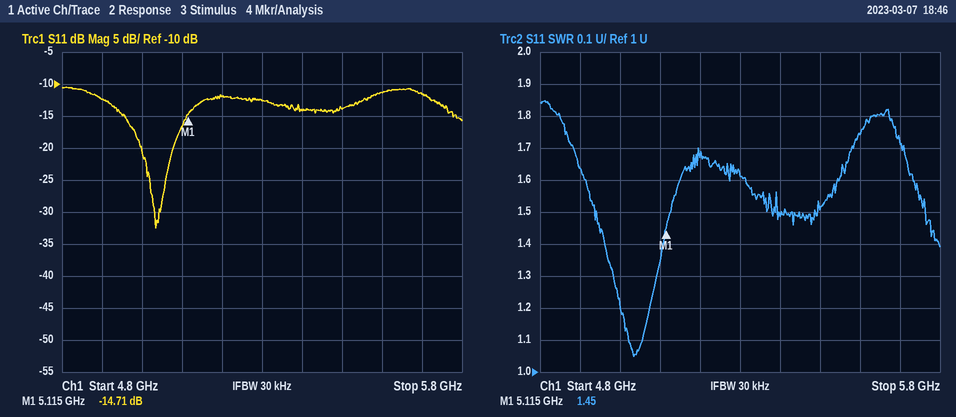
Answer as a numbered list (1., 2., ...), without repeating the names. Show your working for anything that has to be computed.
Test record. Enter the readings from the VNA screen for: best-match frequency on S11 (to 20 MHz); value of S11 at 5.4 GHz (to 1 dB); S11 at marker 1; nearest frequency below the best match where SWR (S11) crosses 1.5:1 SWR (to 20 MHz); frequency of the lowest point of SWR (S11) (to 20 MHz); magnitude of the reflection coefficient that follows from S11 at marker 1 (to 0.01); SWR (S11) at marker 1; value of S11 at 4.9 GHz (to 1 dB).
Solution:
1. 5.04 GHz
2. -14 dB
3. -14.71 dB
4. 4.94 GHz
5. 5.04 GHz
6. 10^(-14.71/20) ≈ 0.18
7. 1.45
8. -12 dB
